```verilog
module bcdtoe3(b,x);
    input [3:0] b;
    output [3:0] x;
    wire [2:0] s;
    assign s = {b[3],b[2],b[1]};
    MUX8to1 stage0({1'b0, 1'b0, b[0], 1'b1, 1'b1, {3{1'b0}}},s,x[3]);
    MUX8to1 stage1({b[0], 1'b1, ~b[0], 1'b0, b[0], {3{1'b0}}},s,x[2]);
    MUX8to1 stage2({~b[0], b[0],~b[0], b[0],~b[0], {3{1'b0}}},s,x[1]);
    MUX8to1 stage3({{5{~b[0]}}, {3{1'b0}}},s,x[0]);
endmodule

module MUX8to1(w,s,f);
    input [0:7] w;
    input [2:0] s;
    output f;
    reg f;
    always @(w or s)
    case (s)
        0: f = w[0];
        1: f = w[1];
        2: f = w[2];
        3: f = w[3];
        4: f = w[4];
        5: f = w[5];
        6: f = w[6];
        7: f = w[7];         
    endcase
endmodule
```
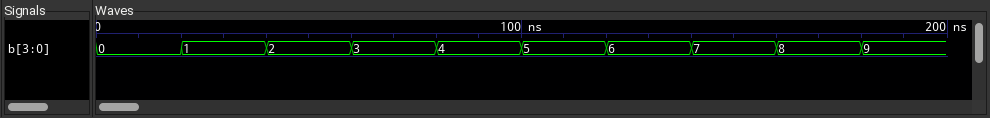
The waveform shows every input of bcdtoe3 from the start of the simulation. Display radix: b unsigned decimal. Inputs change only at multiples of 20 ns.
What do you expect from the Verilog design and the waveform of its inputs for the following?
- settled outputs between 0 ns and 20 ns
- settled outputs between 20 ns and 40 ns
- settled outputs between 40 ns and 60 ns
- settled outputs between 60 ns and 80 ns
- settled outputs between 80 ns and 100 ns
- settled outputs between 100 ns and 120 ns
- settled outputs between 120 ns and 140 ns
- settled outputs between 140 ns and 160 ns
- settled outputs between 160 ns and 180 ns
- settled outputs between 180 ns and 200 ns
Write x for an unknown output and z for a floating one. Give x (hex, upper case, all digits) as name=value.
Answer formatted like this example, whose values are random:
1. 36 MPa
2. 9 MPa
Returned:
1. x=3
2. x=4
3. x=5
4. x=6
5. x=7
6. x=8
7. x=9
8. x=A
9. x=B
10. x=C
